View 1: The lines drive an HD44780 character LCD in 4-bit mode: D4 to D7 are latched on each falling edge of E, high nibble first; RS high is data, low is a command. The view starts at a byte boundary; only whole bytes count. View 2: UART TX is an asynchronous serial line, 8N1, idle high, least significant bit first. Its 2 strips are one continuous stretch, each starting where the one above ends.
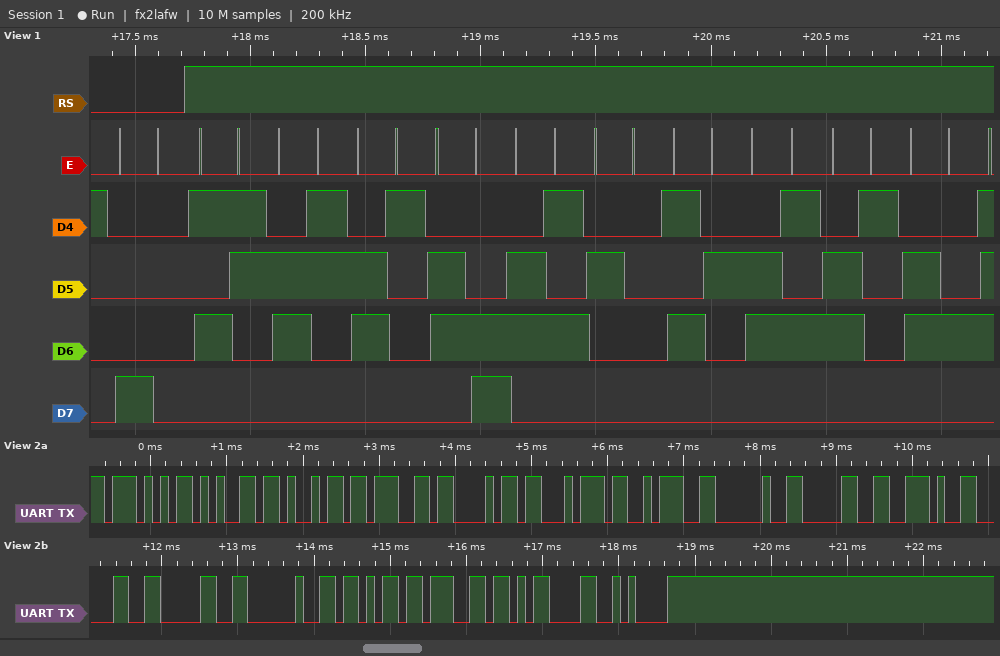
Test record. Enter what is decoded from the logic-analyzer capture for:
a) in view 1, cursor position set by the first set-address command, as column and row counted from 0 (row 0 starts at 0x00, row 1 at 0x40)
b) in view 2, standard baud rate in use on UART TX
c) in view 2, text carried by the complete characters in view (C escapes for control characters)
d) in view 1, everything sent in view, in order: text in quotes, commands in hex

column 0, row 0
9600 baud
"Weight: 0.00 kg\r\n"
0x80 "Scale Read"
